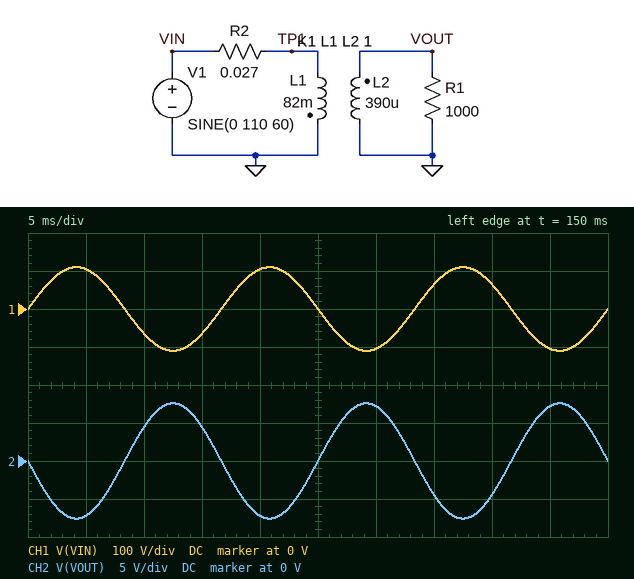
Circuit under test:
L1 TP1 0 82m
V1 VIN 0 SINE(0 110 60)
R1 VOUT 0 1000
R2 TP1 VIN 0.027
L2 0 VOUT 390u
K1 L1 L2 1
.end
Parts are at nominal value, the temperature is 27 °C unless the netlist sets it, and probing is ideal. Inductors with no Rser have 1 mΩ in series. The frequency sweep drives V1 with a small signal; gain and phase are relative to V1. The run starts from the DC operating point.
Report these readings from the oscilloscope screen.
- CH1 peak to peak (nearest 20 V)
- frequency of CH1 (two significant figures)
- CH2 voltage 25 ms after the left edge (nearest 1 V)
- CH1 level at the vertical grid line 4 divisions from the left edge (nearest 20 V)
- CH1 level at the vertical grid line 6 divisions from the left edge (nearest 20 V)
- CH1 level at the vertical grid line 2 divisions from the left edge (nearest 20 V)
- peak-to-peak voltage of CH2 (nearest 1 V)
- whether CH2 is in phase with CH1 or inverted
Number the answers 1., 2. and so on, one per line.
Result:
1. 220 V
2. 60 Hz
3. 0 V
4. 100 V
5. -100 V
6. -60 V
7. 15 V
8. inverted
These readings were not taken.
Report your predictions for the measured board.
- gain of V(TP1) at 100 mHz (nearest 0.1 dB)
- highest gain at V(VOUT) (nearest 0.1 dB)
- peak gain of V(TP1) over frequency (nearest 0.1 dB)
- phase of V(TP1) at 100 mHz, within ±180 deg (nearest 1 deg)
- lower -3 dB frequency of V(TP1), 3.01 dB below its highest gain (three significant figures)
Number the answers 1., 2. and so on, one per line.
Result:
1. -1.1 dB
2. -23.2 dB
3. 0 dB
4. 27 deg
5. 54.3 mHz
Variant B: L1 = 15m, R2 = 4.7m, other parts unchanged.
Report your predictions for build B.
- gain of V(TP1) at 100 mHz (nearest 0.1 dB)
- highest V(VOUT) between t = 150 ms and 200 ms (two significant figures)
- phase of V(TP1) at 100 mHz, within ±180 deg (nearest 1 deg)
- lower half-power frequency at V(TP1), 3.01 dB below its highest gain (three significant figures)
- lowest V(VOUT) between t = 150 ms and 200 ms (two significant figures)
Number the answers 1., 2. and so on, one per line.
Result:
1. -1.3 dB
2. 18 V
3. 25 deg
4. 58.6 mHz
5. -18 V
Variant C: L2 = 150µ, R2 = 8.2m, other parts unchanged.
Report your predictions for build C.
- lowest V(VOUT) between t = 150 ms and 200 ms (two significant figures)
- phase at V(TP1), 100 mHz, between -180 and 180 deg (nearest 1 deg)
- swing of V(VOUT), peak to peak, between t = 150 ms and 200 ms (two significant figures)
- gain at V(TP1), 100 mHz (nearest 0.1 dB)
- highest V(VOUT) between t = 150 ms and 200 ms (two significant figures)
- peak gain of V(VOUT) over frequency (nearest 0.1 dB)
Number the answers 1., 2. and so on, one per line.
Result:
1. -4.7 V
2. 9 deg
3. 9.4 V
4. -0.1 dB
5. 4.7 V
6. -27.4 dB
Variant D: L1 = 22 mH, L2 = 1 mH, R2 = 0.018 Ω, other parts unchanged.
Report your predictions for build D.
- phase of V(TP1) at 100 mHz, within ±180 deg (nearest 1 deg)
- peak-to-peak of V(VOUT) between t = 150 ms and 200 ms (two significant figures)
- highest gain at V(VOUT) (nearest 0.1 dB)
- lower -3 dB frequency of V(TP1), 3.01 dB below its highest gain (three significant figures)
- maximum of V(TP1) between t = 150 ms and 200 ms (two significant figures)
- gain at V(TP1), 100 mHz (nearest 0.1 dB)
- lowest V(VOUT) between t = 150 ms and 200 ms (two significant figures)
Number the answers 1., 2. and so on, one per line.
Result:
1. 50 deg
2. 47 V
3. -13.4 dB
4. 137 mHz
5. 110 V
6. -4.6 dB
7. -23 V
